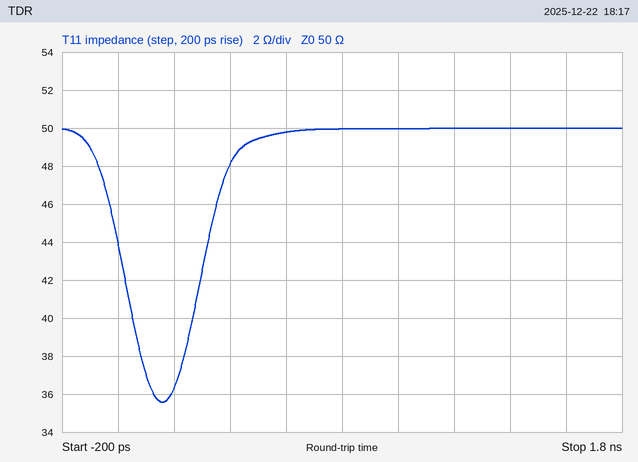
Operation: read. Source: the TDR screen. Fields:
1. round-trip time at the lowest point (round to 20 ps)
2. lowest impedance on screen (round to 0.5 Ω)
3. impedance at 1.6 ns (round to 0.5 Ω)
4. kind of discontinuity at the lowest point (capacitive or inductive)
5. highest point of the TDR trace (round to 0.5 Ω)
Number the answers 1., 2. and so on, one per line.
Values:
1. 160 ps
2. 35.5 Ω
3. 50.0 Ω
4. capacitive
5. 50.0 Ω
